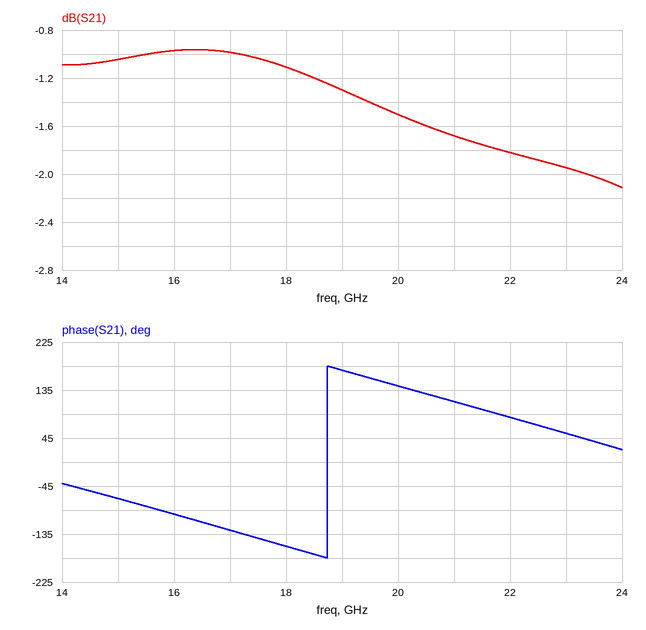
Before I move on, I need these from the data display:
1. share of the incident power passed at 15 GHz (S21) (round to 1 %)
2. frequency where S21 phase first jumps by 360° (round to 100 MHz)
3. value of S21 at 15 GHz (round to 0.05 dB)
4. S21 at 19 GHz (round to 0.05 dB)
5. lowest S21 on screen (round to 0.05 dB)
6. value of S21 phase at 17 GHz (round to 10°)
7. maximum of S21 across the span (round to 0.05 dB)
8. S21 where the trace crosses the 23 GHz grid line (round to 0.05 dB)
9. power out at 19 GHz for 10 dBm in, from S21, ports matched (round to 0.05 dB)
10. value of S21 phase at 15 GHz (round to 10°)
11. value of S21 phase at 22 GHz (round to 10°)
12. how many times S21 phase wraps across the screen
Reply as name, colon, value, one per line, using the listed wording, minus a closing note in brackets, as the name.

share of the incident power passed at 15 GHz (S21): 79 %
frequency where S21 phase first jumps by 360°: 18.7 GHz
value of S21 at 15 GHz: -1.05 dB
S21 at 19 GHz: -1.30 dB
lowest S21 on screen: -2.10 dB
value of S21 phase at 17 GHz: -130°
maximum of S21 across the span: -0.95 dB
S21 where the trace crosses the 23 GHz grid line: -1.95 dB
power out at 19 GHz for 10 dBm in, from S21, ports matched: 8.70 dBm
value of S21 phase at 15 GHz: -70°
value of S21 phase at 22 GHz: 80°
how many times S21 phase wraps across the screen: 1
